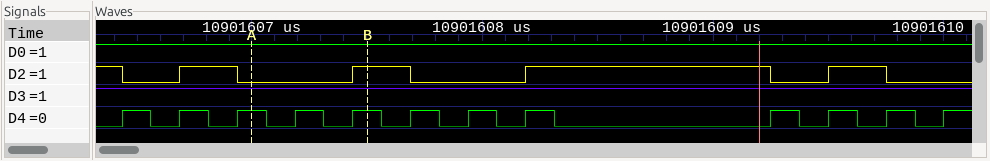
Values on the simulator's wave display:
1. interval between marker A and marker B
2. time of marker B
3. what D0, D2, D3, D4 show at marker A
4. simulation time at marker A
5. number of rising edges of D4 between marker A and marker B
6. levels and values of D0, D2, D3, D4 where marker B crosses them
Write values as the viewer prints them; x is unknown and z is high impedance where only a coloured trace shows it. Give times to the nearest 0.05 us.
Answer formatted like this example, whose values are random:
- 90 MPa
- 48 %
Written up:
- 0.5 us
- 10901607.5 us
- D0=1, D2=0, D3=1, D4=1
- 10901607 us
- 2
- D0=1, D2=1, D3=1, D4=1
